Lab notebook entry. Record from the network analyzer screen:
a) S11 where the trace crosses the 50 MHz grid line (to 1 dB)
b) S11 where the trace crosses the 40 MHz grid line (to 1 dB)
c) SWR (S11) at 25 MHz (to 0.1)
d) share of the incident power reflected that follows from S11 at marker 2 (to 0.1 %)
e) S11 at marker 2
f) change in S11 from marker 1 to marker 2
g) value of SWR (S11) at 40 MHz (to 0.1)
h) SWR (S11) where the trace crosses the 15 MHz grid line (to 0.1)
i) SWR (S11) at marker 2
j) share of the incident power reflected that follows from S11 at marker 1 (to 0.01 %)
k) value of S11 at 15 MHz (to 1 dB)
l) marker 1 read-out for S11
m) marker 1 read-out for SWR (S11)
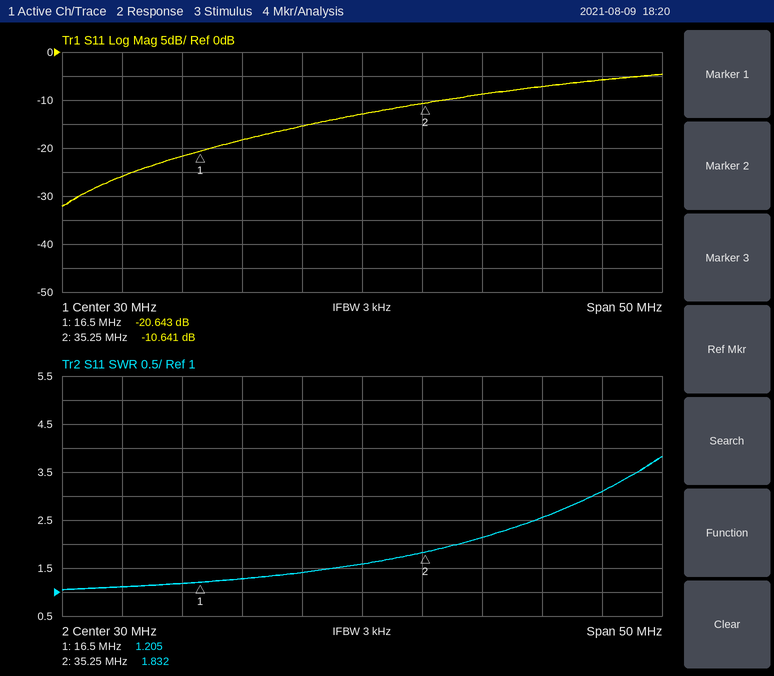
-6 dB
-9 dB
1.4
8.6 %
-10.641 dB
10.002 dB
2.1
1.2
1.832
0.86 %
-22 dB
-20.643 dB
1.205
